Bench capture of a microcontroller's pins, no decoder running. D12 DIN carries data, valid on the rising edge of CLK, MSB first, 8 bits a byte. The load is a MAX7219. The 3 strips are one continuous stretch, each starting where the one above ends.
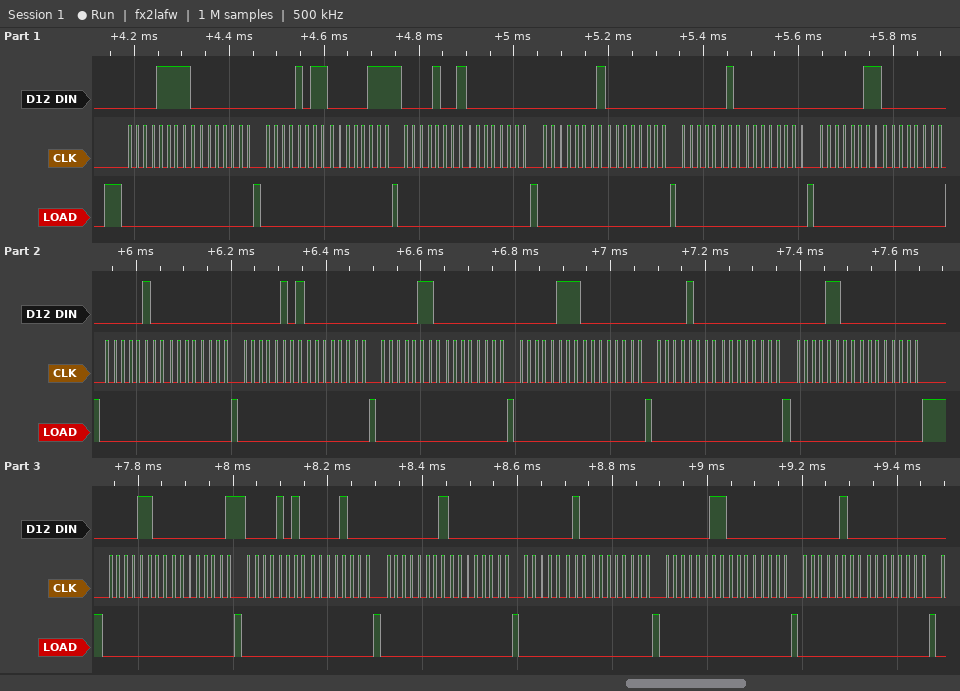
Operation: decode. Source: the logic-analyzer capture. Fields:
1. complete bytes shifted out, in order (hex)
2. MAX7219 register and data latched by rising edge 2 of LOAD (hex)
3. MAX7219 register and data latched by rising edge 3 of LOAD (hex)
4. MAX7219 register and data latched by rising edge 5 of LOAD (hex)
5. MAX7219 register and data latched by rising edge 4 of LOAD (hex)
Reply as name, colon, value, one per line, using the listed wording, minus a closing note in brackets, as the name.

complete bytes shifted out, in order: 0x0F 0x00 0x0B 0x07 0x09 0x00 0x01 0x00 0x02 0x00 0x03 0x00 0x04 0x00 0x05 0x00 0x06 0x00 0x07 0x00 0x08 0x00 0x0C 0x00 0x0C 0x01 0x0A 0x08 0x01 0x00 0x02 0x00 0x03 0x00 0x04 0x00
MAX7219 register and data latched by rising edge 2 of LOAD: register 0xF, data 0x00
MAX7219 register and data latched by rising edge 3 of LOAD: register 0xB, data 0x07
MAX7219 register and data latched by rising edge 5 of LOAD: register 0x1, data 0x00
MAX7219 register and data latched by rising edge 4 of LOAD: register 0x9, data 0x00
